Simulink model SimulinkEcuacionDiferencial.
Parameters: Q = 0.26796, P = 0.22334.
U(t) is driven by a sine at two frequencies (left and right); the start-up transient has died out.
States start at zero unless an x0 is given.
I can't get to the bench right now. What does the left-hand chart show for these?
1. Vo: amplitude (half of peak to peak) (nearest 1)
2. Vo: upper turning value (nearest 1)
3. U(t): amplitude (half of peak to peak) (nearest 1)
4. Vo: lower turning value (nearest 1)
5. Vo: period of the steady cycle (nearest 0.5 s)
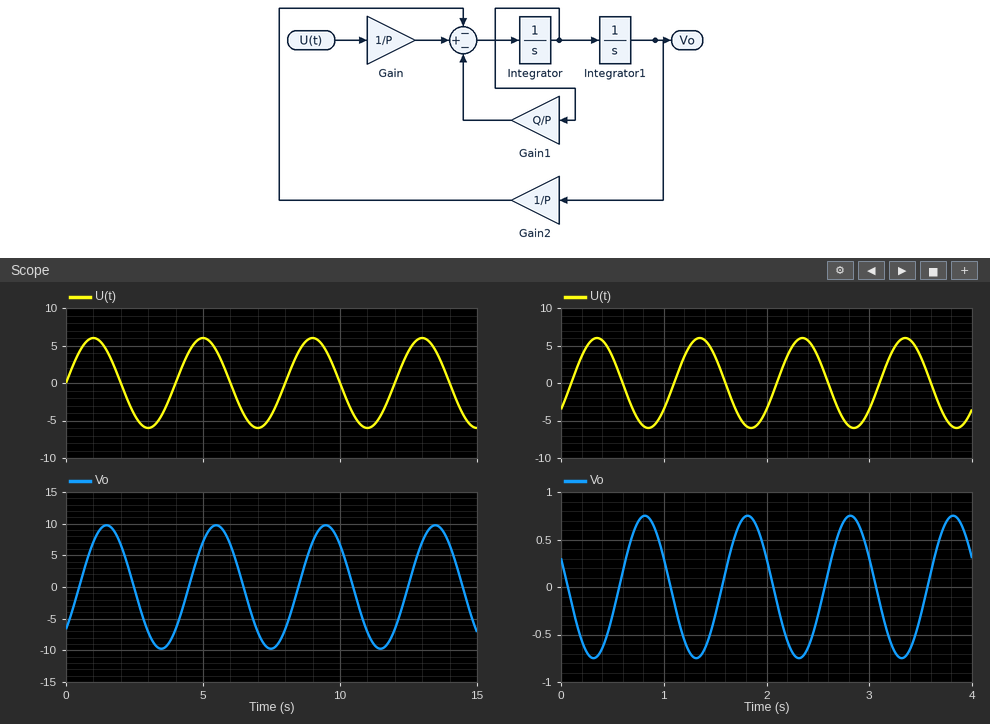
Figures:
10
10
6
-10
4.0 s
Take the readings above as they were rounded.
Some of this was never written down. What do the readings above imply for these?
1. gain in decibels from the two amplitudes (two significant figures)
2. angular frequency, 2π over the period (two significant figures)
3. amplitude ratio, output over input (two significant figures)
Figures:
4.4 dB
1.6 rad/s
1.7
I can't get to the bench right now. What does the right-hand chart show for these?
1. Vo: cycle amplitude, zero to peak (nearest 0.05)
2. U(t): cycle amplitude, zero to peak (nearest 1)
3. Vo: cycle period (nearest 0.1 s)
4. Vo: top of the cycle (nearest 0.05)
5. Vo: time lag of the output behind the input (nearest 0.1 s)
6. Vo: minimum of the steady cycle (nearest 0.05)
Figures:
0.75
6
1.0 s
0.75
0.5 s
-0.75
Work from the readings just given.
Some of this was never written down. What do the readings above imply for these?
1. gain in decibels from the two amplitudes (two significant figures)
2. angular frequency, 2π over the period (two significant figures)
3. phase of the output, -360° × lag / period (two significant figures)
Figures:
-18 dB
6.3 rad/s
-180°
